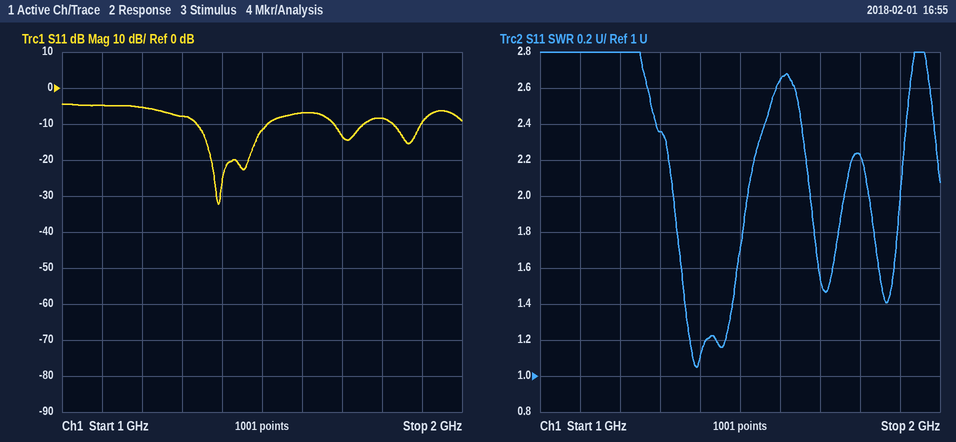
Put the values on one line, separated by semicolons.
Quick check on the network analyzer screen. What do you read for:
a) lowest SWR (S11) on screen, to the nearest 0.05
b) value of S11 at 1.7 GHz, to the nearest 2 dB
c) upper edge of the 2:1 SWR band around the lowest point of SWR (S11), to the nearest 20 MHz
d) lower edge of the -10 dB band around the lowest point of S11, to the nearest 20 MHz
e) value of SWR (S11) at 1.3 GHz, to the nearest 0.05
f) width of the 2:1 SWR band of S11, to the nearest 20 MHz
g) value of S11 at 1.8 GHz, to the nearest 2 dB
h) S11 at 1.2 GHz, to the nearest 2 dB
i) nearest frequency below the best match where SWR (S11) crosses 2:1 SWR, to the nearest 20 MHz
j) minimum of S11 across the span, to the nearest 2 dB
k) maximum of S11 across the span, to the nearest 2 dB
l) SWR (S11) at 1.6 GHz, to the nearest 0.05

1.05; -14 dB; 1.52 GHz; 1.34 GHz; 2.35; 180 MHz; -8 dB; -6 dB; 1.34 GHz; -32 dB; -4 dB; 2.65
